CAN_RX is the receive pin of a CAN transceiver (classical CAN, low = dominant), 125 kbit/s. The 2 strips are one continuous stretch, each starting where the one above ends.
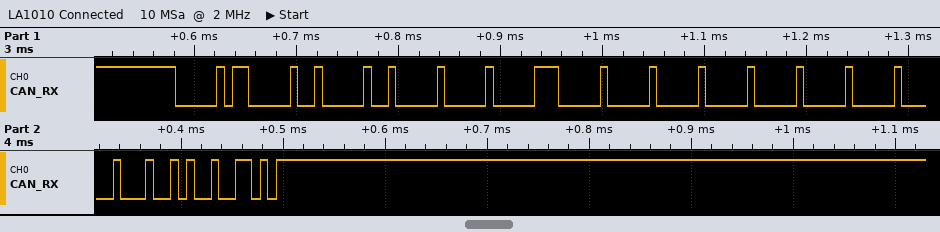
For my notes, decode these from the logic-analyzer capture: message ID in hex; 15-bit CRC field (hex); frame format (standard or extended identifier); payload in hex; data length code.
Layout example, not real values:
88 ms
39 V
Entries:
0x030
0x2526
standard
08 00 0C 00 00 00 00 00
8
